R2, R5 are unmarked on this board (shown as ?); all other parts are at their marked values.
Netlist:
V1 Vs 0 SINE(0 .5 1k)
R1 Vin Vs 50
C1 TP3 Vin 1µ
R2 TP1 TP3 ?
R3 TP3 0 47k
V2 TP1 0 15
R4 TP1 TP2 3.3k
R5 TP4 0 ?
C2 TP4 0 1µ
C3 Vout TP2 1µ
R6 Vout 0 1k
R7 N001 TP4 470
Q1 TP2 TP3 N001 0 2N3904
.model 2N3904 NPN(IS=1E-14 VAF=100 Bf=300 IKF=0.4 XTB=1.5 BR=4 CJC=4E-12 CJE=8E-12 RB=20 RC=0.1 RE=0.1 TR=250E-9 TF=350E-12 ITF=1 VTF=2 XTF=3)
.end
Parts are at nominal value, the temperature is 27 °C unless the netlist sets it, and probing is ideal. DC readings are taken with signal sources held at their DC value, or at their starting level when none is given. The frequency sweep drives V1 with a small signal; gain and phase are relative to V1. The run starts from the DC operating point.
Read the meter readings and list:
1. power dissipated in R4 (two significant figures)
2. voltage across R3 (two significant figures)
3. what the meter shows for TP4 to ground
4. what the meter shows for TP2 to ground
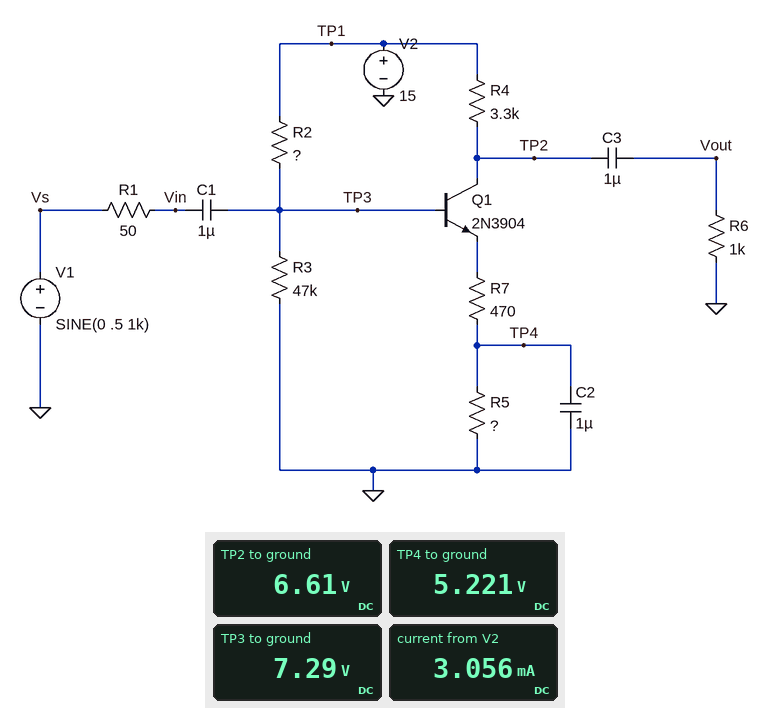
21 mW
7.3 V
5.221 V
6.61 V
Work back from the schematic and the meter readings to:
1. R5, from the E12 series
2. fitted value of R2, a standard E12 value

1.8 kΩ
15 kΩ
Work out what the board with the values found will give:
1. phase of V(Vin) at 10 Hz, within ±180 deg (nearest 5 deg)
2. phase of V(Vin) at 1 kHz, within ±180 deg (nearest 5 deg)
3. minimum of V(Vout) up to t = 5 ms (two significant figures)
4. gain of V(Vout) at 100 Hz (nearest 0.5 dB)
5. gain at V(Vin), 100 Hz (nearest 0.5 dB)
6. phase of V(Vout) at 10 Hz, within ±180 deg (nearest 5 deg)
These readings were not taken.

0 deg
-5 deg
-390 mV
-15.5 dB
0 dB
165 deg
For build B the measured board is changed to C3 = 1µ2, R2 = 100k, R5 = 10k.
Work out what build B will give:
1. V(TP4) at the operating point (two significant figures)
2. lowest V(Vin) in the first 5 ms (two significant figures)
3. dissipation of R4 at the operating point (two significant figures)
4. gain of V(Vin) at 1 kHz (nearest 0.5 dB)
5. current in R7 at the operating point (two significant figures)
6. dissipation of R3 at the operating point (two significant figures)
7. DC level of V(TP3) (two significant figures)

3.9 V
-500 mV
510 µW
0 dB
390 µA
480 µW
4.8 V
